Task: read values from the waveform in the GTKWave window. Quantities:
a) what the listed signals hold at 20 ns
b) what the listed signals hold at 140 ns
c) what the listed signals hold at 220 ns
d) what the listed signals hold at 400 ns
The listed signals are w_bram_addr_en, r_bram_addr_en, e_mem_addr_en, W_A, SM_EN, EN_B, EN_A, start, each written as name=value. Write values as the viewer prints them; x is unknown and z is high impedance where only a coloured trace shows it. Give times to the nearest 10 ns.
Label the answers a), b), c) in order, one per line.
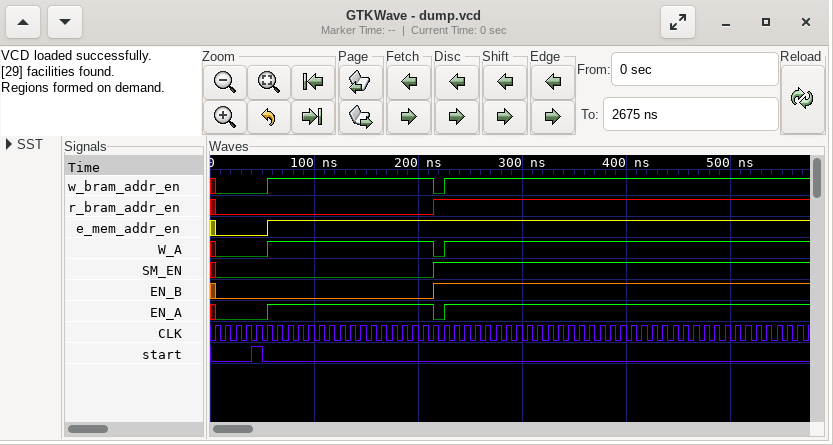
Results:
a) w_bram_addr_en=0, r_bram_addr_en=0, e_mem_addr_en=0, W_A=0, SM_EN=0, EN_B=0, EN_A=0, start=0
b) w_bram_addr_en=1, r_bram_addr_en=0, e_mem_addr_en=1, W_A=1, SM_EN=0, EN_B=0, EN_A=1, start=0
c) w_bram_addr_en=0, r_bram_addr_en=1, e_mem_addr_en=1, W_A=0, SM_EN=1, EN_B=1, EN_A=0, start=0
d) w_bram_addr_en=1, r_bram_addr_en=1, e_mem_addr_en=1, W_A=1, SM_EN=1, EN_B=1, EN_A=1, start=0
